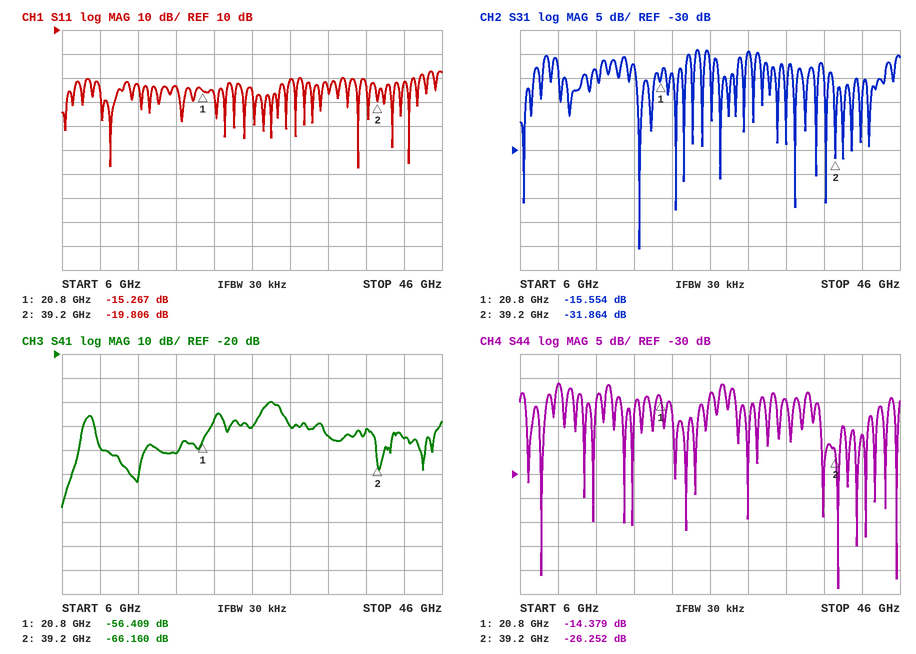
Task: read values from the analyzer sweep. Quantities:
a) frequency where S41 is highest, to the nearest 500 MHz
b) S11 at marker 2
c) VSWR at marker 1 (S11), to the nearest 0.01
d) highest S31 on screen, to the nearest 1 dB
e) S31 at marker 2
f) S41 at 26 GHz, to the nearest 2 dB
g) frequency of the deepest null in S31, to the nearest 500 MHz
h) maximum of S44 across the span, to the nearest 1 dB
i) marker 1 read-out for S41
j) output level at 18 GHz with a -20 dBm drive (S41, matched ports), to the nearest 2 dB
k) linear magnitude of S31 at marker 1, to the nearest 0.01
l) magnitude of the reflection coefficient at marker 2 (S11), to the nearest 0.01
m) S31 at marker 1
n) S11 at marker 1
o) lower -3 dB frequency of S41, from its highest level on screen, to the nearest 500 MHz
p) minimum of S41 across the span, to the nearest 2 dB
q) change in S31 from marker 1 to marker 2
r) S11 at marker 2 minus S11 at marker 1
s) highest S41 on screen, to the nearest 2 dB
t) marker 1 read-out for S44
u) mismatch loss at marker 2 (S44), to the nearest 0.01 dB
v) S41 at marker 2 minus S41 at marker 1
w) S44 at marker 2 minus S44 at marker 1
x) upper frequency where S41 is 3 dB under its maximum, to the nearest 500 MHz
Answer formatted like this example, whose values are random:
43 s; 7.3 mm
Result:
28.0 GHz; -19.806 dB; 1.42; -9 dB; -31.864 dB; -50 dB; 18.5 GHz; -11 dB; -56.409 dB; -82 dBm; 0.17; 0.10; -15.554 dB; -15.267 dB; 27.0 GHz; -84 dB; -16.310 dB; -4.539 dB; -40 dB; -14.379 dB; 0.01 dB; -9.751 dB; -11.873 dB; 29.0 GHz
